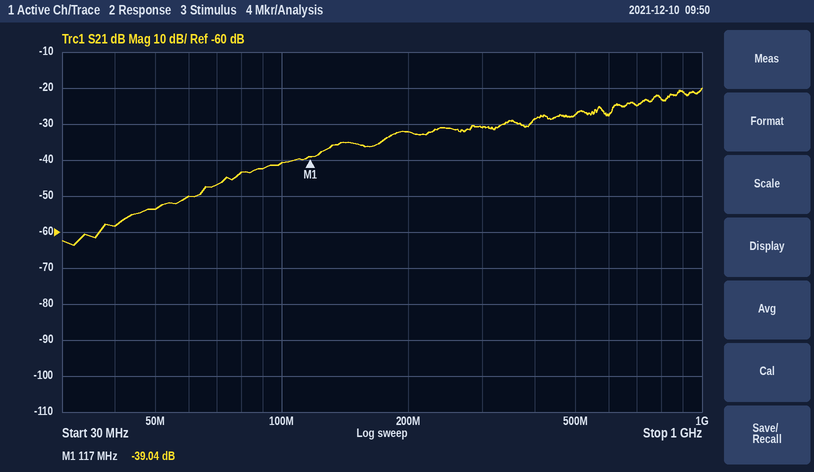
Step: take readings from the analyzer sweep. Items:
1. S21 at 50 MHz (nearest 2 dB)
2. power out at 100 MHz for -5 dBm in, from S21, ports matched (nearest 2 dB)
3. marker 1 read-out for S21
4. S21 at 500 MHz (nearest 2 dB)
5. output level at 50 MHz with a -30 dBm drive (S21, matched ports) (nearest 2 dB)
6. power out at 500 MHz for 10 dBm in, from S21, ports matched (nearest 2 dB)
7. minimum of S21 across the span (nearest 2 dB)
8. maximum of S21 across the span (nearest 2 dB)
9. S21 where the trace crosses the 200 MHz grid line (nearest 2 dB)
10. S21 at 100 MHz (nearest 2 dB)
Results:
-54 dB
-46 dBm
-39.04 dB
-28 dB
-84 dBm
-18 dBm
-64 dB
-20 dB
-32 dB
-40 dB
